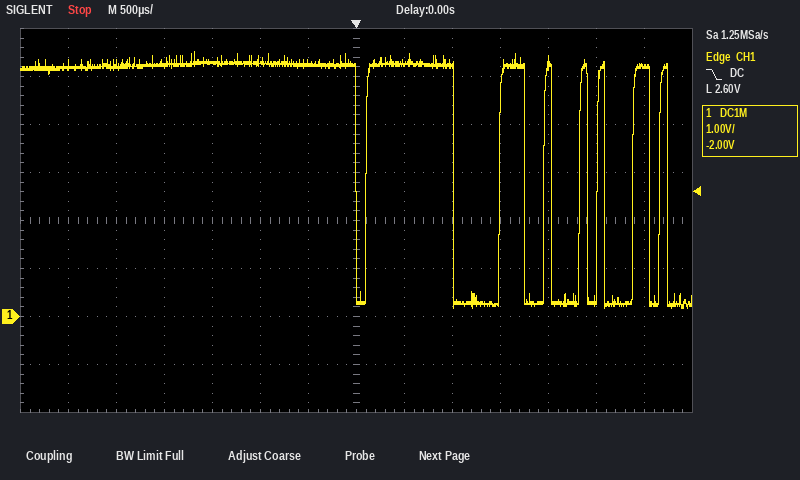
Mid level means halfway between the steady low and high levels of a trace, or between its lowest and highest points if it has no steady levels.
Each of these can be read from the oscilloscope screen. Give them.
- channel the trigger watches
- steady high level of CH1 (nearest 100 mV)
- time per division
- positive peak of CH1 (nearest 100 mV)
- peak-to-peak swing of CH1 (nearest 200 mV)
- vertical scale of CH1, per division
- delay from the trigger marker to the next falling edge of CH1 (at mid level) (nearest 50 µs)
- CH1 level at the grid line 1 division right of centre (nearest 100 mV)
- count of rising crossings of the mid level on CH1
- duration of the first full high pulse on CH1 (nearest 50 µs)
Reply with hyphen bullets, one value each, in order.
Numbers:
- CH1
- 5.2 V
- 500 µs
- 5.5 V
- 5.4 V
- 1 V
- 1.00 ms
- 5.3 V
- 7
- 900 µs
